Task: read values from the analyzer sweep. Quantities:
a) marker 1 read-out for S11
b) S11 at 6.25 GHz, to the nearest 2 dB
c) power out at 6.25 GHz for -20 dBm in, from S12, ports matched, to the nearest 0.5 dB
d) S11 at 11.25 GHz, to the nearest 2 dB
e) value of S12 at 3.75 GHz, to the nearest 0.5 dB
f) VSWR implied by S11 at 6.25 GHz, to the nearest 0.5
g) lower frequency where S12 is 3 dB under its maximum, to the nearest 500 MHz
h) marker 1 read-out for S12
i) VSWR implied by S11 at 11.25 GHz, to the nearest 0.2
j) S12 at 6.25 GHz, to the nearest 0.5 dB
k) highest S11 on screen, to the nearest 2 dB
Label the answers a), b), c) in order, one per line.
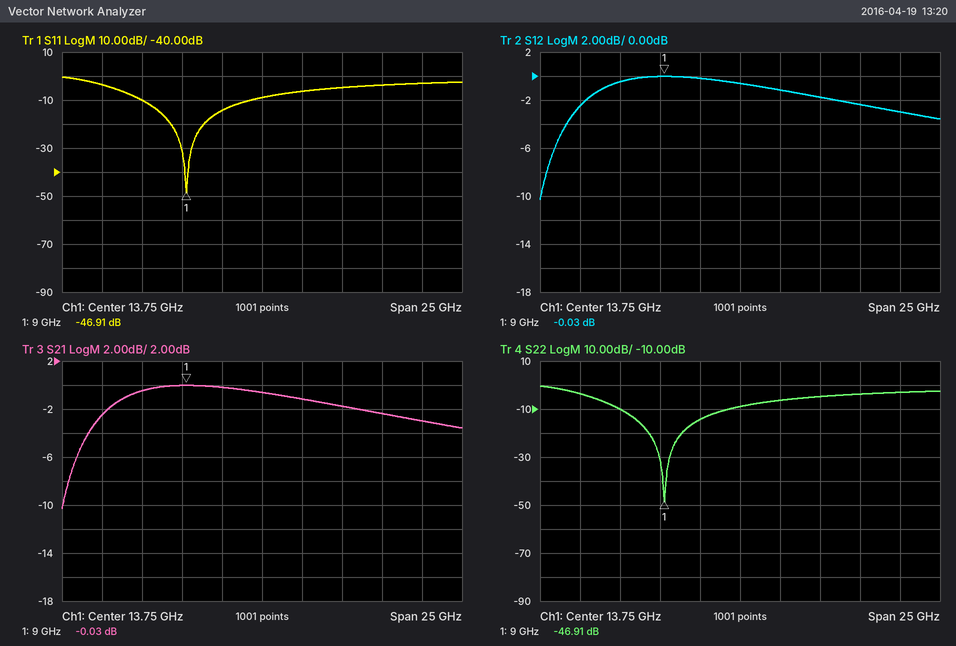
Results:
a) -46.91 dB
b) -10 dB
c) -20.5 dBm
d) -14 dB
e) -2.5 dB
f) 2.0
g) 3.5 GHz
h) -0.03 dB
i) 1.4
j) -0.5 dB
k) 0 dB
